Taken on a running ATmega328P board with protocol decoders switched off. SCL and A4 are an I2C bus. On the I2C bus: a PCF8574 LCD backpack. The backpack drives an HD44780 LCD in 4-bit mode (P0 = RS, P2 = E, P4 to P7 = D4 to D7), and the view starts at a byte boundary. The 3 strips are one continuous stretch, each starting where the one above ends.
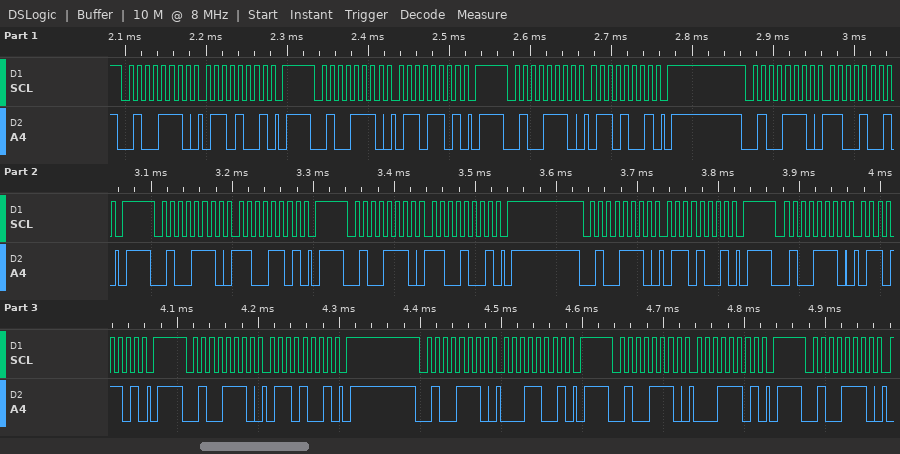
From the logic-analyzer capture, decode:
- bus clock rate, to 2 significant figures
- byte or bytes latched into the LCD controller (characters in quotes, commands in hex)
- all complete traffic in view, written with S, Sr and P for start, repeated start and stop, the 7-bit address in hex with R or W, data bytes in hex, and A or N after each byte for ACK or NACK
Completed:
100 kHz
'l'
S 27W A 69 A P S 27W A 6D A P S 27W A 69 A P S 27W A C9 A P S 27W A CD A P S 27W A C9 A P S 27W A 69 A P S 27W A 6D A P S 27W A 69 A P S 27W A 19 A P S 27W A 1D A P S 27W A
